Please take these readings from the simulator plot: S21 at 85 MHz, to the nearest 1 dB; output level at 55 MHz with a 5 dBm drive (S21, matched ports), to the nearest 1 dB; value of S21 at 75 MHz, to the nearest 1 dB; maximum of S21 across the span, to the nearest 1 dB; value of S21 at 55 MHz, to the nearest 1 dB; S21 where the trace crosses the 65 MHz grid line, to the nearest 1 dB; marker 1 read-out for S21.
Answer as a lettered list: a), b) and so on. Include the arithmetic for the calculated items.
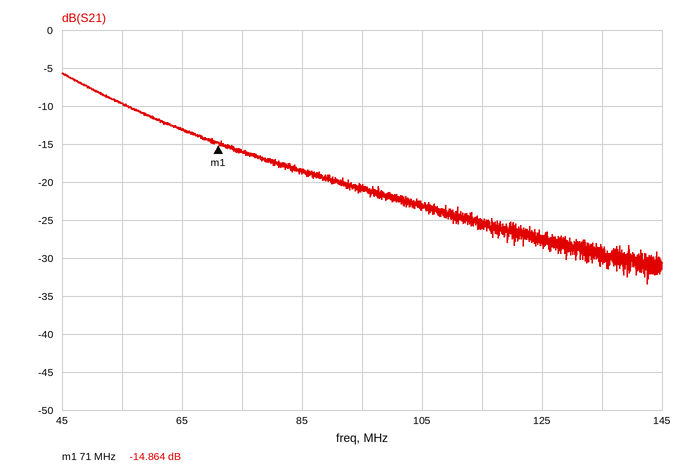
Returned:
a) -19 dB
b) 5 dBm + (-10 dB) = -5 dBm
c) -16 dB
d) -6 dB
e) -10 dB
f) -13 dB
g) -14.864 dB
